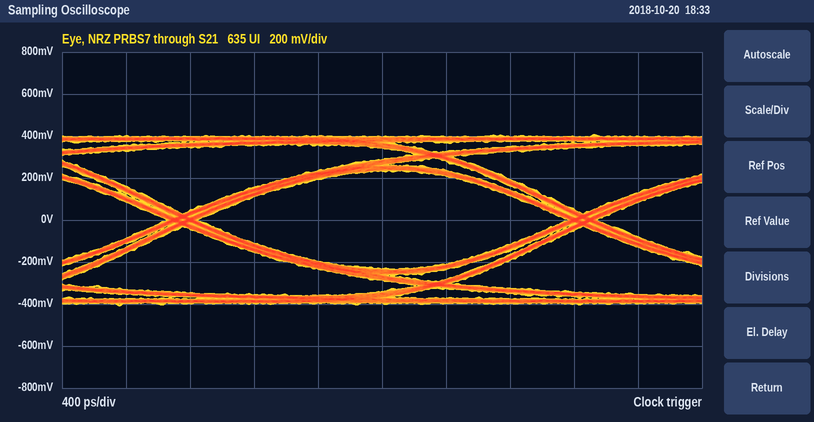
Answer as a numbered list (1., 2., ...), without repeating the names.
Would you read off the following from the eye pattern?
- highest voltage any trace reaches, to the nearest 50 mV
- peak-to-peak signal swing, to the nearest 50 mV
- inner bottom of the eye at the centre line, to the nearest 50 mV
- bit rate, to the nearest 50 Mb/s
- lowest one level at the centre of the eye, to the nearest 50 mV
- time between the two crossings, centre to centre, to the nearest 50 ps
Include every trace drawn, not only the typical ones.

1. 400 mV
2. 800 mV
3. -250 mV
4. 400 Mb/s
5. 250 mV
6. 2.50 ns
